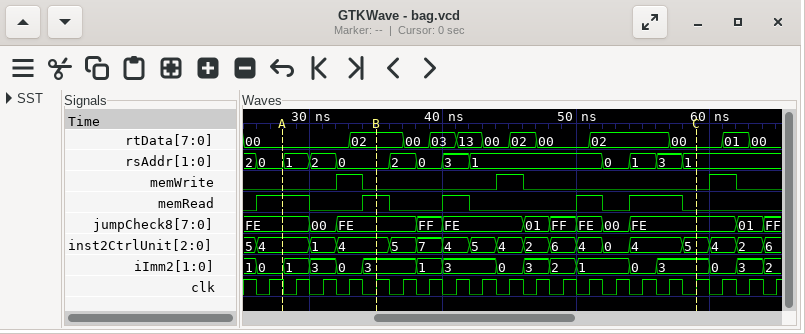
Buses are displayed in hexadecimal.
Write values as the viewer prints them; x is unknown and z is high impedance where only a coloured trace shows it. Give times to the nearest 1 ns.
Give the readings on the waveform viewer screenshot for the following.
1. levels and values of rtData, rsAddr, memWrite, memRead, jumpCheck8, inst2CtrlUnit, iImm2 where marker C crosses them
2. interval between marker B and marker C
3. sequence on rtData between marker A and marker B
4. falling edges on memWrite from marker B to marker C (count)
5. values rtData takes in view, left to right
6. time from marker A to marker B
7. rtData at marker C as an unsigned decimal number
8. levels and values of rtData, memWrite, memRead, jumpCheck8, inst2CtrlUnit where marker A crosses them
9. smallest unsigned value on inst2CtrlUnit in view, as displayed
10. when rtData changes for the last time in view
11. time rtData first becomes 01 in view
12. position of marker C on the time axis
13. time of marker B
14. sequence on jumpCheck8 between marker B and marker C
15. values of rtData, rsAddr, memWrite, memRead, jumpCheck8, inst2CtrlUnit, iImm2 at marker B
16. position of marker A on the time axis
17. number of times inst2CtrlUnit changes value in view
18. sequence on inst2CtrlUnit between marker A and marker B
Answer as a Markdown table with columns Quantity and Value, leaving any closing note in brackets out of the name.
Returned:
| Quantity | Value |
|---|---|
| levels and values of rtData, rsAddr, memWrite, memRead, jumpCheck8, inst2CtrlUnit, iImm2 where marker C crosses them | rtData=00, rsAddr=1, memWrite=0, memRead=0, jumpCheck8=FE, inst2CtrlUnit=5, iImm2=3 |
| interval between marker B and marker C | 24 ns |
| sequence on rtData between marker A and marker B | 00, 02 |
| falling edges on memWrite from marker B to marker C | 1 |
| values rtData takes in view, left to right | 00, 02, 00, 03, 13, 00, 02, 00, 02, 00, 01, 00 |
| time from marker A to marker B | 7 ns |
| rtData at marker C as an unsigned decimal number | 0 |
| levels and values of rtData, memWrite, memRead, jumpCheck8, inst2CtrlUnit where marker A crosses them | rtData=00, memWrite=0, memRead=1, jumpCheck8=FE, inst2CtrlUnit=4 |
| smallest unsigned value on inst2CtrlUnit in view, as displayed | 0 |
| when rtData changes for the last time in view | 63 ns |
| time rtData first becomes 01 in view | 61 ns |
| position of marker C on the time axis | 59 ns |
| time of marker B | 35 ns |
| sequence on jumpCheck8 between marker B and marker C | FE, FF, FE, 01, FF, FE, 00, FE |
| values of rtData, rsAddr, memWrite, memRead, jumpCheck8, inst2CtrlUnit, iImm2 at marker B | rtData=02, rsAddr=0, memWrite=0, memRead=1, jumpCheck8=FE, inst2CtrlUnit=4, iImm2=3 |
| position of marker A on the time axis | 28 ns |
| number of times inst2CtrlUnit changes value in view | 17 |
| sequence on inst2CtrlUnit between marker A and marker B | 4, 1, 4 |
